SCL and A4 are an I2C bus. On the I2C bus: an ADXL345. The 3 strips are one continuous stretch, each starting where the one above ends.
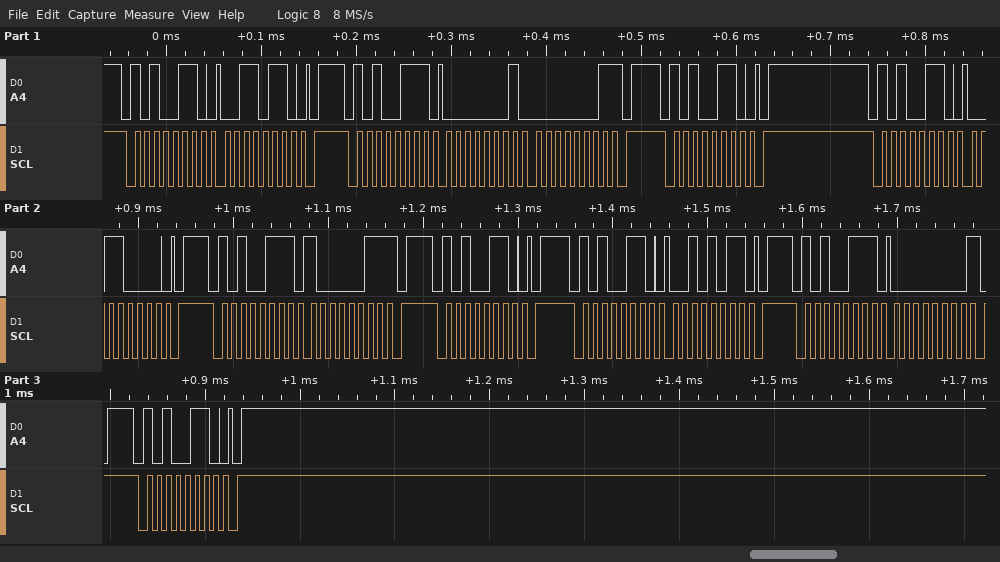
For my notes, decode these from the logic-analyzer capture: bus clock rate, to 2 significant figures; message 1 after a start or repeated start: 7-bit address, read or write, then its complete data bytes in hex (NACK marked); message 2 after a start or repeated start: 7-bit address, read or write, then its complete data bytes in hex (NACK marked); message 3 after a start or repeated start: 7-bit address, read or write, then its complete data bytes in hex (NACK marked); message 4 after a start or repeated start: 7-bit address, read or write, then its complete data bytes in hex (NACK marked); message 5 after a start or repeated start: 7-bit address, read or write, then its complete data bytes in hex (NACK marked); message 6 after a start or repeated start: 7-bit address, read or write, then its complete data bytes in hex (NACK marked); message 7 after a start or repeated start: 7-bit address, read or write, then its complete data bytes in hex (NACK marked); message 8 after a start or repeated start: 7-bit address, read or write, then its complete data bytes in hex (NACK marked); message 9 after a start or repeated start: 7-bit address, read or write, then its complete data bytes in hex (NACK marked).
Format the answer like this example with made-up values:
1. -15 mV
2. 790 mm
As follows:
1. 100 kHz
2. 0x53 write: 36
3. 0x53 read: 01 01 NACK
4. 0x53 write
5. 0x53 write: 30
6. 0x53 read: 83 NACK
7. 0x53 write
8. 0x53 write: 2B
9. 0x53 read: 00 NACK
10. 0x53 write
